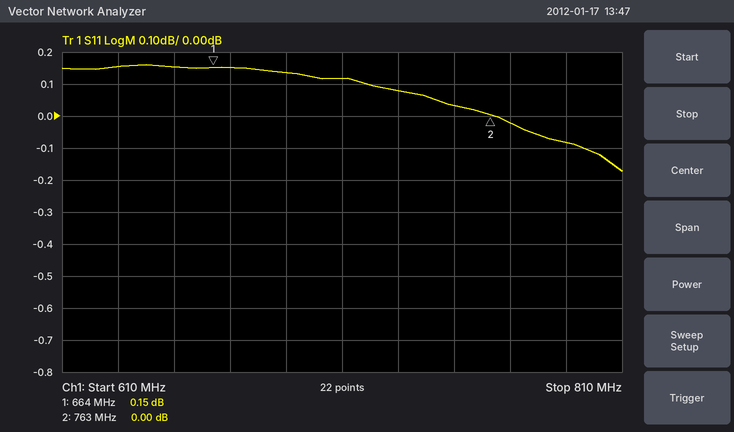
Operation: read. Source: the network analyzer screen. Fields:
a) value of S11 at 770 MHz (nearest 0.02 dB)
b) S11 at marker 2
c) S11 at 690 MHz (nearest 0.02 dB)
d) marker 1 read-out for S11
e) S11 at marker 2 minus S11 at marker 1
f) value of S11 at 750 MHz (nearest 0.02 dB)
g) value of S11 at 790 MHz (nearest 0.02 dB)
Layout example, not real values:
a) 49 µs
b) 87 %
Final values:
a) -0.02 dB
b) 0.00 dB
c) 0.14 dB
d) 0.15 dB
e) -0.15 dB
f) 0.04 dB
g) -0.08 dB
